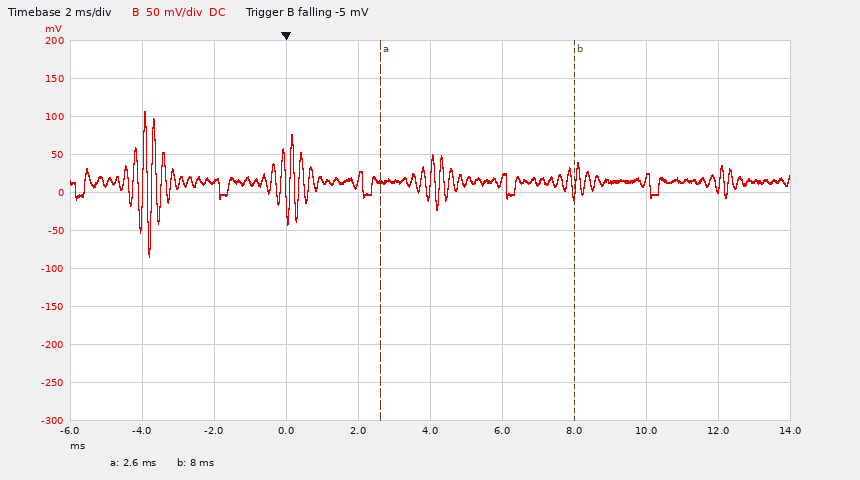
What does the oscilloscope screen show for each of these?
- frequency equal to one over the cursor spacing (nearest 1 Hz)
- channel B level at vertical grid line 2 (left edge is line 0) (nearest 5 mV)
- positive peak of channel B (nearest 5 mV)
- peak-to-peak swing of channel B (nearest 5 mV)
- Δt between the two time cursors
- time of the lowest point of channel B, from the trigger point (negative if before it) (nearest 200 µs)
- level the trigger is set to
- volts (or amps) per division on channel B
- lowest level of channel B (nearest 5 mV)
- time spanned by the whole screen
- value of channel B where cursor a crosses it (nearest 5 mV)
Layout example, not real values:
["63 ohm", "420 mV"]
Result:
["185 Hz", "15 mV", "105 mV", "190 mV", "5.4 ms", "-3.8 ms", "-5 mV", "50 mV", "-85 mV", "20 ms", "15 mV"]
